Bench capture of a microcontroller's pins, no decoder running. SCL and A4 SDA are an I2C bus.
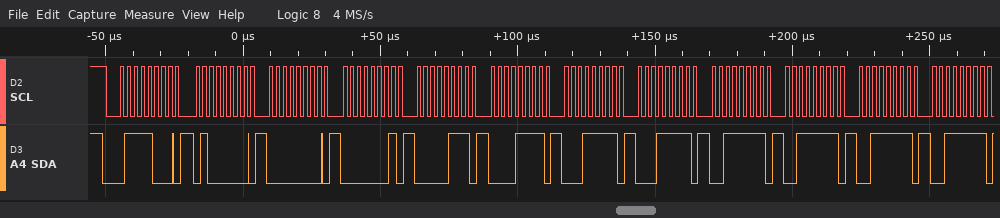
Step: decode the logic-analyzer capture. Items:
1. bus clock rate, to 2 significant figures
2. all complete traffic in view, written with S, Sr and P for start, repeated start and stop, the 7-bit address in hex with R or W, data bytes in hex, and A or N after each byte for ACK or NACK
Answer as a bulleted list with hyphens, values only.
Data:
- 400 kHz
- S 3CW A 40 A 00 A 01 A 07 A 0F A 1F A 1F A 3F A 3F A 3F A 3F A
